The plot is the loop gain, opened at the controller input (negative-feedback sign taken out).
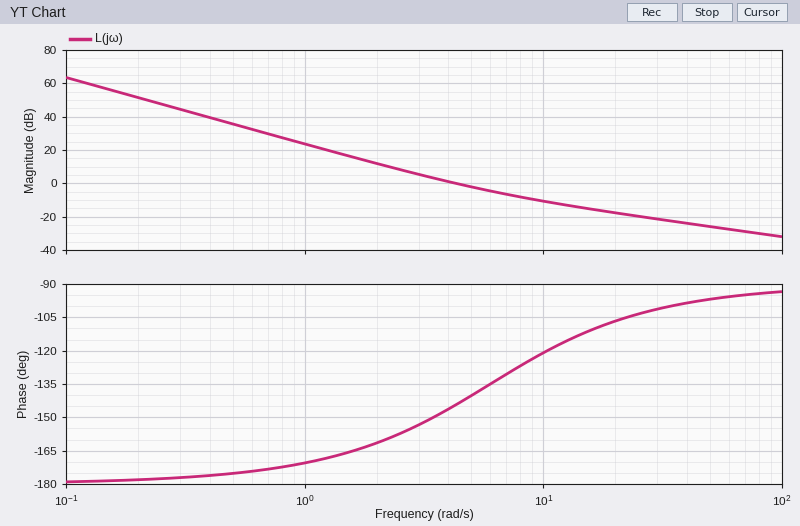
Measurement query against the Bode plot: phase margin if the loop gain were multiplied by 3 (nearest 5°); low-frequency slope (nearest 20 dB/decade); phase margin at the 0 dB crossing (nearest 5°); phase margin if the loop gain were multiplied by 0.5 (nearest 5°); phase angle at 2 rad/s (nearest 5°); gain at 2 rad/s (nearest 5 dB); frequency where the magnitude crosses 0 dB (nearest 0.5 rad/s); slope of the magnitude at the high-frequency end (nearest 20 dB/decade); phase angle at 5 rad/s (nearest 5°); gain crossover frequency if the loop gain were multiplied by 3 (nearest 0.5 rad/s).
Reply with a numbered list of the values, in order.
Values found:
1. 55°
2. -40 dB/decade
3. 35°
4. 25°
5. -160°
6. 10 dB
7. 4.5 rad/s
8. -20 dB/decade
9. -140°
10. 9.0 rad/s
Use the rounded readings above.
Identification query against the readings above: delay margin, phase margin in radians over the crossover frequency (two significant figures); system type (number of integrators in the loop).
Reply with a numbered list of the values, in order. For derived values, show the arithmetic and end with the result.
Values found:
1. 35 × π / 180 / 4.5 = 0.14 s
2. 2
